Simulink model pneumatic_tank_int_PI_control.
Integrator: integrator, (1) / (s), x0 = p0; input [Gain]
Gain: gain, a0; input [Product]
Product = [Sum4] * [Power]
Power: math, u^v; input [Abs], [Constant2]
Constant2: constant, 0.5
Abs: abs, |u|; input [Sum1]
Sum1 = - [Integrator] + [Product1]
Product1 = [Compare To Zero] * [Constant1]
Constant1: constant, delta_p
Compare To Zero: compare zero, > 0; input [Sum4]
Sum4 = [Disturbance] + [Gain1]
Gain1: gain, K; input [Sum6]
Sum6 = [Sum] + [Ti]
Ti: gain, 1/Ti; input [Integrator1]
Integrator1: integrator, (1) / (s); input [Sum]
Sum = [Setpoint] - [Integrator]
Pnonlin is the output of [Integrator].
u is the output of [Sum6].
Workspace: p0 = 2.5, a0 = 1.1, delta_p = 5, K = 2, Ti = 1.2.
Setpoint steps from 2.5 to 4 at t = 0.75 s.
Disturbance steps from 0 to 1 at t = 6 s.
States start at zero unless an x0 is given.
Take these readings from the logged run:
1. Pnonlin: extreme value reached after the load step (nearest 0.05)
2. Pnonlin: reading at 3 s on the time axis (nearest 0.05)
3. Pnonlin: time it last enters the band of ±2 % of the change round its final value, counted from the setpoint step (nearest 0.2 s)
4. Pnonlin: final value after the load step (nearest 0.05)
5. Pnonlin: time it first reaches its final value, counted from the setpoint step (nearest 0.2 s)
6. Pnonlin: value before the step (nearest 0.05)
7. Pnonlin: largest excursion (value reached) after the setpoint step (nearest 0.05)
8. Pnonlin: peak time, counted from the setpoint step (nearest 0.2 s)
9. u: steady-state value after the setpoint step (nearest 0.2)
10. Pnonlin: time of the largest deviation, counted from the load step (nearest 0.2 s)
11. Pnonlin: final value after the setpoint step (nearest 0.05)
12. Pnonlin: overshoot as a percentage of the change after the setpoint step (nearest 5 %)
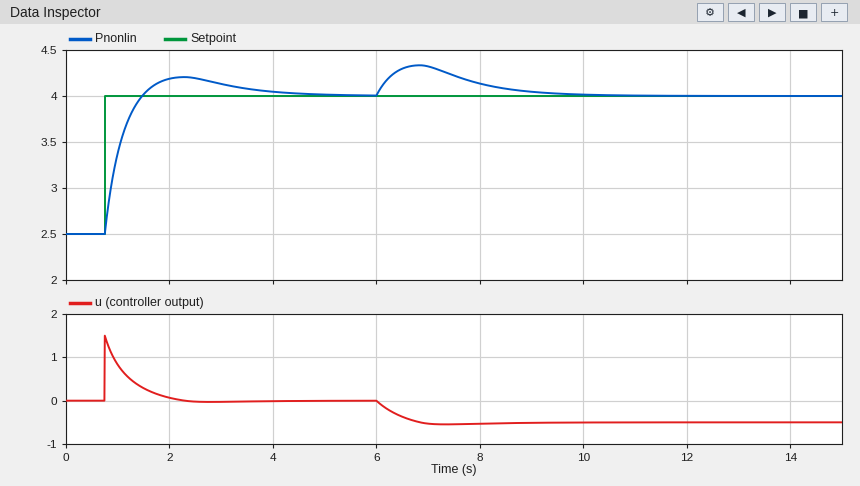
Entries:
4.35
4.15
3.6 s
4.00
0.8 s
2.50
4.20
1.6 s
0.0
0.8 s
4.00
15 %
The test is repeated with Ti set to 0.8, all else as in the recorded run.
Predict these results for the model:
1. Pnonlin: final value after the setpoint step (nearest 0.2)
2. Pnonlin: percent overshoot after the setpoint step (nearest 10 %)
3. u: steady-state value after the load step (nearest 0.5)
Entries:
4.0
20 %
-0.5
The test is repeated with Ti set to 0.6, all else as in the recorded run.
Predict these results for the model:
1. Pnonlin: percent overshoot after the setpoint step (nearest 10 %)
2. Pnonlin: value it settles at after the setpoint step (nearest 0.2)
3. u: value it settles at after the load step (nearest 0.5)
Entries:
20 %
4.0
-0.5
